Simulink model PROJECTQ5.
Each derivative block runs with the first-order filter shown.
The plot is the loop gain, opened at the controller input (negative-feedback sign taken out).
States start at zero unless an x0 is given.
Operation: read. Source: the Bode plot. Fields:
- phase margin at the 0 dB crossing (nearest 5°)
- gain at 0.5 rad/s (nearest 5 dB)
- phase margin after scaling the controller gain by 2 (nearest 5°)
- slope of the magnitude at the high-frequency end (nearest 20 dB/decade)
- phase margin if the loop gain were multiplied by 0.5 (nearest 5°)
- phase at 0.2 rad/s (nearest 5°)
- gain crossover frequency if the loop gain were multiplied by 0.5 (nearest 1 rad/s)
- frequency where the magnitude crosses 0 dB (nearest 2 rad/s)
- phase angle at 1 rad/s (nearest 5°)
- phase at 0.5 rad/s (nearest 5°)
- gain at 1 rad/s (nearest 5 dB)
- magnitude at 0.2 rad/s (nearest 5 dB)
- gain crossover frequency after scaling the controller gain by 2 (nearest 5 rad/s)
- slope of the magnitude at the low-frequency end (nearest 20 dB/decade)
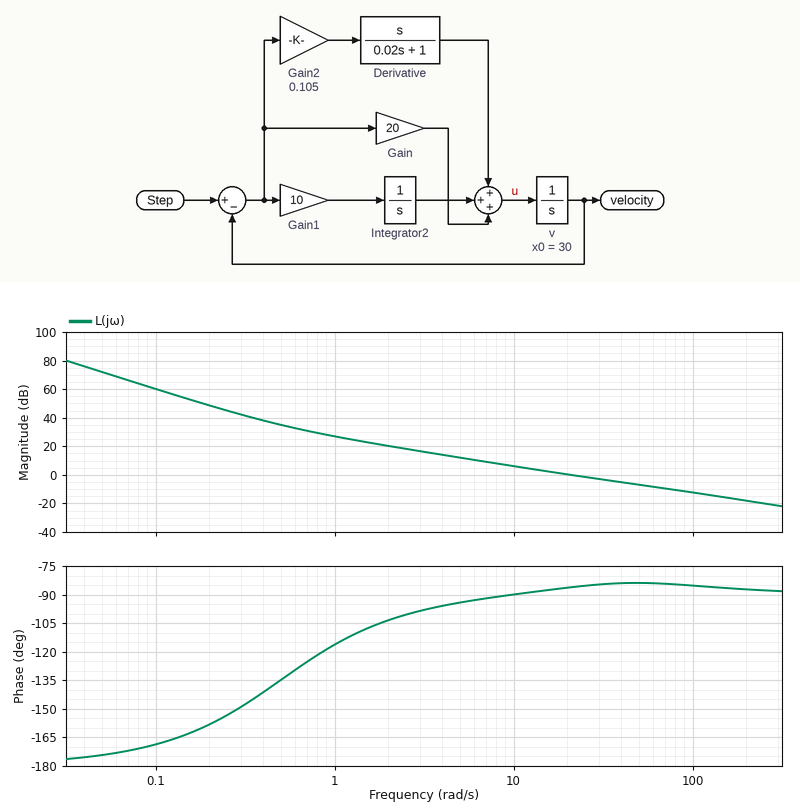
95°
35 dB
95°
-20 dB/decade
90°
-160°
10 rad/s
20 rad/s
-115°
-135°
25 dB
50 dB
45 rad/s
-40 dB/decade
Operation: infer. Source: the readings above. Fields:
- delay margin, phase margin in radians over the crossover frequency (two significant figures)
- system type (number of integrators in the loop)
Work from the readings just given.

0.083 s
2
